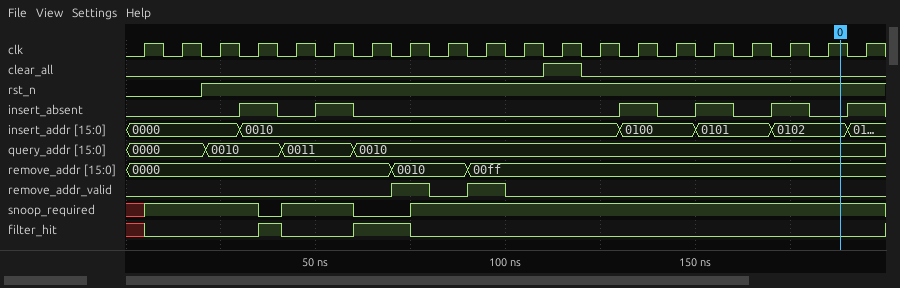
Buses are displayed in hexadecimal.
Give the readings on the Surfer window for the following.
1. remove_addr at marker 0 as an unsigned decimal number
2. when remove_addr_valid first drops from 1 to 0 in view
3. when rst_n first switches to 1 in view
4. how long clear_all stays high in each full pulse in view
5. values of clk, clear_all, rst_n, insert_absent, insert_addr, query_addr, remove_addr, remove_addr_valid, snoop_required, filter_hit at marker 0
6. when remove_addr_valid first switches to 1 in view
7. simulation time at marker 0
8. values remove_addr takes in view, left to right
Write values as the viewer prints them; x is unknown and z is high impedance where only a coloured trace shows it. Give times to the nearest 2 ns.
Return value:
255
80 ns
20 ns
10 ns
clk=1, clear_all=0, rst_n=1, insert_absent=0, insert_addr=0102, query_addr=0010, remove_addr=00ff, remove_addr_valid=0, snoop_required=1, filter_hit=0
70 ns
188 ns
0000, 0010, 00ff
